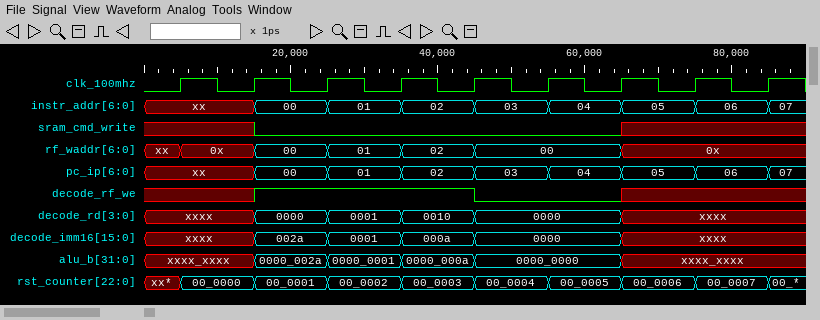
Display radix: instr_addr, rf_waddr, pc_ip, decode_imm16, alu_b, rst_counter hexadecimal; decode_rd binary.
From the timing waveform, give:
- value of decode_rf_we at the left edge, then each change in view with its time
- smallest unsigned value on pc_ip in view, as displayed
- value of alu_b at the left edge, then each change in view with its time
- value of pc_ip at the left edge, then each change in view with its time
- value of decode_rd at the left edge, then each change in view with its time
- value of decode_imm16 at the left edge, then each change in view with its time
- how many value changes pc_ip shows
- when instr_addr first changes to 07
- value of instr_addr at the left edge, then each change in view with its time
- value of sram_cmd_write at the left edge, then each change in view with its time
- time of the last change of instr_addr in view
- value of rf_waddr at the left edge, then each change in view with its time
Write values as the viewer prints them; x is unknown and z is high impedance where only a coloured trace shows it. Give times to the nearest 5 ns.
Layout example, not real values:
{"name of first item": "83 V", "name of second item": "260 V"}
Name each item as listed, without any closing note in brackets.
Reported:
{"value of decode_rf_we at the left edge, then each change in view with its time": "x, 1 at 15 ns, 0 at 45 ns, x at 65 ns", "smallest unsigned value on pc_ip in view, as displayed": "00", "value of alu_b at the left edge, then each change in view with its time": "xxxx_xxxx, 0000_002a at 15 ns, 0000_0001 at 25 ns, 0000_000a at 35 ns, 0000_0000 at 45 ns, xxxx_xxxx at 65 ns", "value of pc_ip at the left edge, then each change in view with its time": "xx, 00 at 15 ns, 01 at 25 ns, 02 at 35 ns, 03 at 45 ns, 04 at 55 ns, 05 at 65 ns, 06 at 75 ns, 07 at 85 ns", "value of decode_rd at the left edge, then each change in view with its time": "xxxx, 0000 at 15 ns, 0001 at 25 ns, 0010 at 35 ns, 0000 at 45 ns, xxxx at 65 ns", "value of decode_imm16 at the left edge, then each change in view with its time": "xxxx, 002a at 15 ns, 0001 at 25 ns, 000a at 35 ns, 0000 at 45 ns, xxxx at 65 ns", "how many value changes pc_ip shows": "8", "when instr_addr first changes to 07": "85 ns", "value of instr_addr at the left edge, then each change in view with its time": "xx, 00 at 15 ns, 01 at 25 ns, 02 at 35 ns, 03 at 45 ns, 04 at 55 ns, 05 at 65 ns, 06 at 75 ns, 07 at 85 ns", "value of sram_cmd_write at the left edge, then each change in view with its time": "x, 0 at 15 ns, x at 65 ns", "time of the last change of instr_addr in view": "85 ns", "value of rf_waddr at the left edge, then each change in view with its time": "xx, 0x at 5 ns, 00 at 15 ns, 01 at 25 ns, 02 at 35 ns, 00 at 45 ns, 0x at 65 ns"}
